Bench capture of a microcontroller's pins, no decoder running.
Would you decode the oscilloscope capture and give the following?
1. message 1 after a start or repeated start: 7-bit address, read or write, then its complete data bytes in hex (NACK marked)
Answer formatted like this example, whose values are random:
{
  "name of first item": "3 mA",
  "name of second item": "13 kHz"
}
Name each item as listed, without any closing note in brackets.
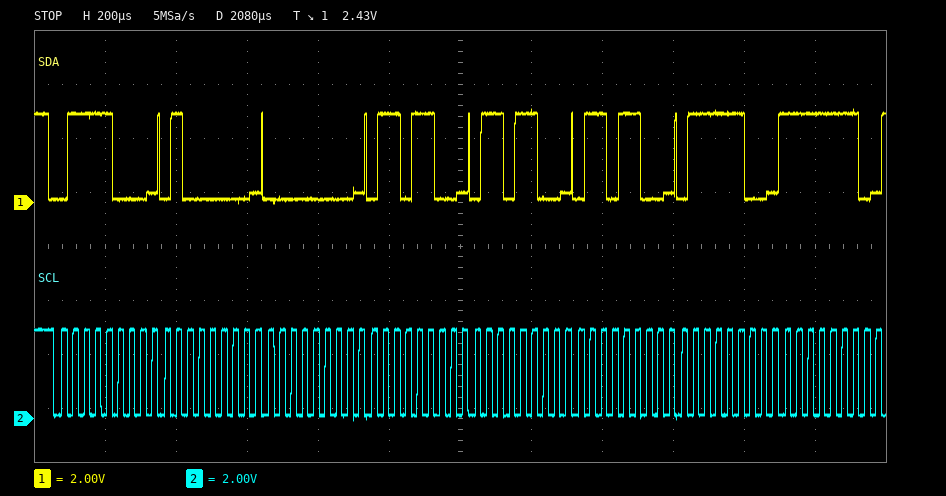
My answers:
{
  "message 1 after a start or repeated start: 7-bit address, read or write, then its complete data bytes in hex": "0x3C write: 40 00 6C 6C 6C 7C FE"
}
